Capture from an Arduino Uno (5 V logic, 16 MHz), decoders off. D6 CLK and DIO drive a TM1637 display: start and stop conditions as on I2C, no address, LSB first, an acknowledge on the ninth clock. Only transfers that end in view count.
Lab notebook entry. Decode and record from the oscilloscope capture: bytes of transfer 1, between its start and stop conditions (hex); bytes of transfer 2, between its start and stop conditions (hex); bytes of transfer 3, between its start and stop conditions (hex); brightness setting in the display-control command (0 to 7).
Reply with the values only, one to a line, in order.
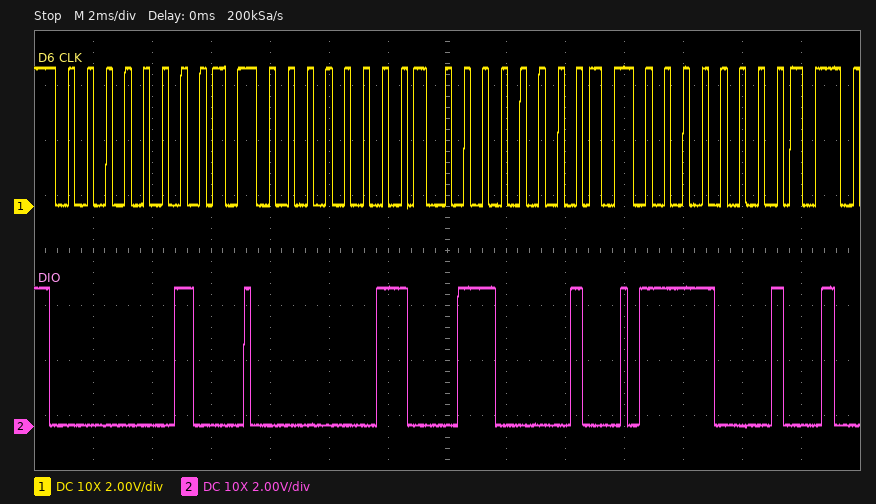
40
C0 86
8F
7
